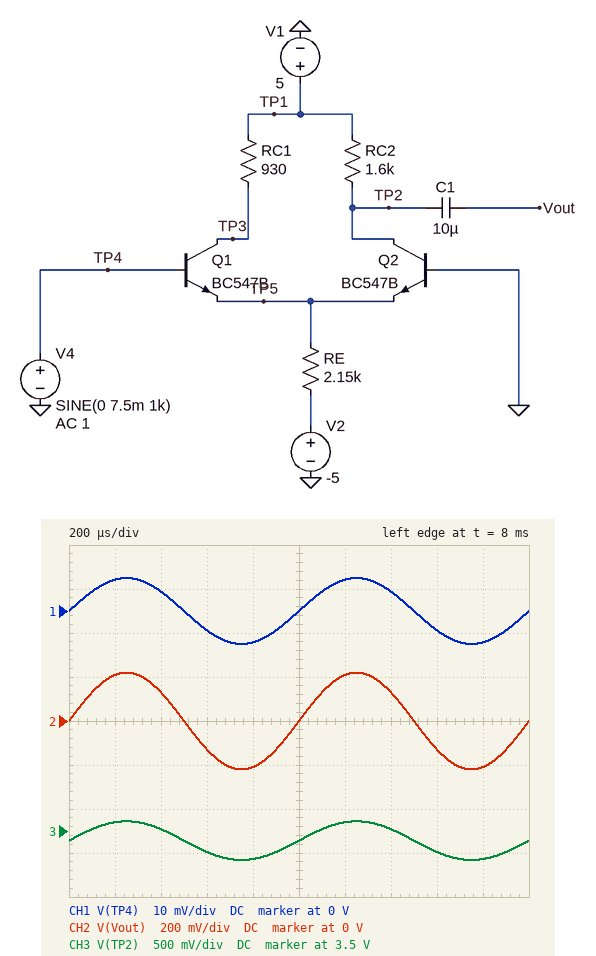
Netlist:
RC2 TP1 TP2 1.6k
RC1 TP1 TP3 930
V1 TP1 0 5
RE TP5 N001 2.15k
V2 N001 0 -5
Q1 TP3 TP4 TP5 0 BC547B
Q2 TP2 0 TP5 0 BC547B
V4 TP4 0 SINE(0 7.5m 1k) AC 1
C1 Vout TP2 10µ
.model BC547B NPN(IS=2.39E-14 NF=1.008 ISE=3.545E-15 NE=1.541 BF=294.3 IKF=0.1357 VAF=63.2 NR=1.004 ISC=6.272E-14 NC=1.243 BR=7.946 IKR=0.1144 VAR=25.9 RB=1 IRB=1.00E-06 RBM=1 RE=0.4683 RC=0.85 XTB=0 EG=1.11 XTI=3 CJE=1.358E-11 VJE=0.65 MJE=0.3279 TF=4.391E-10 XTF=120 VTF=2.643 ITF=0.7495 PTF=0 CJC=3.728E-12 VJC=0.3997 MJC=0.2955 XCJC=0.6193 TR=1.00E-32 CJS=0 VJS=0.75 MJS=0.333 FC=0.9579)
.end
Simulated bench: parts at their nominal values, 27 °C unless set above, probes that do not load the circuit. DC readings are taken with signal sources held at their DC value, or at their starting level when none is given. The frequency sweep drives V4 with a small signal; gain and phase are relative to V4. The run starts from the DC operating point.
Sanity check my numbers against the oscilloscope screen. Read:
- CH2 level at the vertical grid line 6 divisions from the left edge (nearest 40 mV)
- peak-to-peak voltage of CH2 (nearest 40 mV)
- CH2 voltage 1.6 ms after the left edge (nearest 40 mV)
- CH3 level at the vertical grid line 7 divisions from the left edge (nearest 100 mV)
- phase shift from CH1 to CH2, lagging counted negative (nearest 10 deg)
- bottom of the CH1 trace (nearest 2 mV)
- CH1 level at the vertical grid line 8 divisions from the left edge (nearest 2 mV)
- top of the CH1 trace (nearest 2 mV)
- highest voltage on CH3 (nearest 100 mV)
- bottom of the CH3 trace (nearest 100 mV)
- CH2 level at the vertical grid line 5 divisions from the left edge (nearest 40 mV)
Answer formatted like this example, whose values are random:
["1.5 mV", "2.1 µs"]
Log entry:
["200 mV", "440 mV", "-120 mV", "3.5 V", "0 deg", "-8 mV", "-4 mV", "8 mV", "3.6 V", "3.2 V", "0 V"]
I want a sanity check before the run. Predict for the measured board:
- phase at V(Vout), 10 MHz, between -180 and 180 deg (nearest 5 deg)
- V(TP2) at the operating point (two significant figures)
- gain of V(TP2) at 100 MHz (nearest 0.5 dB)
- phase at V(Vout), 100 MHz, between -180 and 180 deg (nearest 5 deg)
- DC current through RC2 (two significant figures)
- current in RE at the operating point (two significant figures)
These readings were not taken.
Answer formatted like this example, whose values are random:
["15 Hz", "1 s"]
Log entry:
["-10 deg", "3.4 V", "22.5 dB", "-65 deg", "1.0 mA", "2.0 mA"]
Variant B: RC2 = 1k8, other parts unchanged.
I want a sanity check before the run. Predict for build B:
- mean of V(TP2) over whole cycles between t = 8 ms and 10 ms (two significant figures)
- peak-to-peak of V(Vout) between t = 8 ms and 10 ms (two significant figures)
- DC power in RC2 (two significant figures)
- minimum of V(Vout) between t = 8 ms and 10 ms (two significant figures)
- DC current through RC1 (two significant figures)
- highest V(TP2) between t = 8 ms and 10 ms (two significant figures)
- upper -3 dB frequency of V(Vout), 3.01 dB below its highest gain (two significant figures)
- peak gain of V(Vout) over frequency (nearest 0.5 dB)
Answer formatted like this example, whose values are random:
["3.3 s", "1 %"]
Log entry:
["3.2 V", "490 mV", "1.8 mW", "-250 mV", "1.0 mA", "3.4 V", "45 MHz", "30.5 dB"]
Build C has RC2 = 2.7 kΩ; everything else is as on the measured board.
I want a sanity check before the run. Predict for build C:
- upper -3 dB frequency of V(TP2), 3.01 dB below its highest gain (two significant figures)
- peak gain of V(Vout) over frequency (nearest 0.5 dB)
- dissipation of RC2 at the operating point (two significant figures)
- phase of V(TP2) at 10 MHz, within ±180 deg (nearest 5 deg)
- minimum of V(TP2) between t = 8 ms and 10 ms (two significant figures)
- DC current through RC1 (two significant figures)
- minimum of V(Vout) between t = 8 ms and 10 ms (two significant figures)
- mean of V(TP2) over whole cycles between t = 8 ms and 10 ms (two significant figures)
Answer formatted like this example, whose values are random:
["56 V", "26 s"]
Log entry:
["28 MHz", "34.0 dB", "2.7 mW", "-20 deg", "1.9 V", "1.0 mA", "-370 mV", "2.3 V"]
